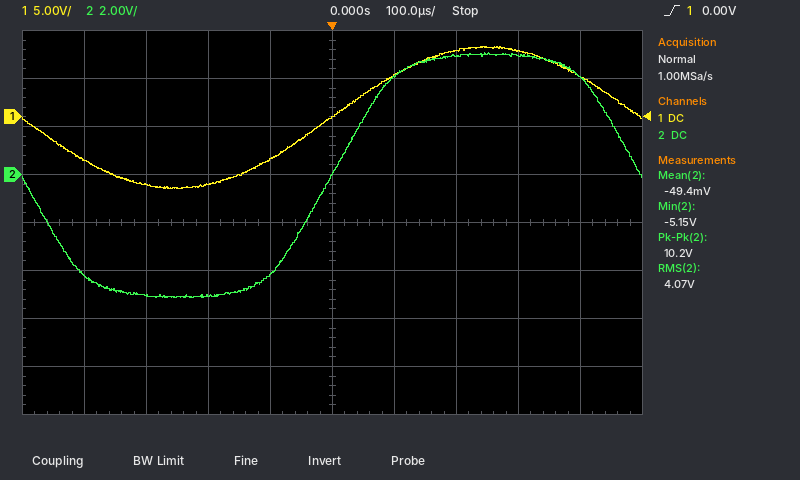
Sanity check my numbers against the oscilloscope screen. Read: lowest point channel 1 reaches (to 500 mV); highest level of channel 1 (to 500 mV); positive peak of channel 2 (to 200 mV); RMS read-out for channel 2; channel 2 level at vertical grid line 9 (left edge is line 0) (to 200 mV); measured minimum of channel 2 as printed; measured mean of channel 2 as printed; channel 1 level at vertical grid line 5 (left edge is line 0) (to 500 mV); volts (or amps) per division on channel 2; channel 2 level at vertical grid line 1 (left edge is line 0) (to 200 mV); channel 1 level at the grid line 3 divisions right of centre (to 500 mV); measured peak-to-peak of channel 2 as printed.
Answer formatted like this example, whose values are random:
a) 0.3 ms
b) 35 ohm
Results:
a) -7.5 V
b) 7.5 V
c) 5.0 V
d) 4.07 V
e) 4.0 V
f) -5.15 V
g) -49.4 mV
h) 0.0 V
i) 2 V
j) -4.2 V
k) 7.0 V
l) 10.2 V
